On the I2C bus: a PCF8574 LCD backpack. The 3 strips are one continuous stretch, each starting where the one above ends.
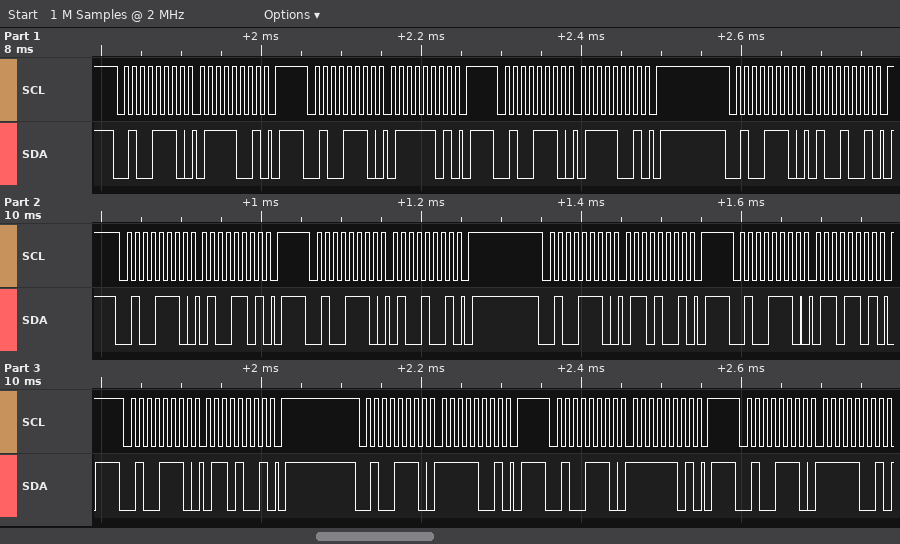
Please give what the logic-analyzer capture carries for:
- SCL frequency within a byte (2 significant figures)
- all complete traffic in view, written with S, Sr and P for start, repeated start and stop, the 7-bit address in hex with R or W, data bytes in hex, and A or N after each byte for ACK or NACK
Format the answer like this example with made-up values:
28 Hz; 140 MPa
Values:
100 kHz; S 27W A 79 A P S 27W A 7D A P S 27W A 79 A P S 27W A 49 A P S 27W A 4D A P S 27W A 49 A P S 27W A 69 A P S 27W A 6D A P S 27W A 69 A P S 27W A F9 A P S 27W A FD A P S 27W A F9 A
